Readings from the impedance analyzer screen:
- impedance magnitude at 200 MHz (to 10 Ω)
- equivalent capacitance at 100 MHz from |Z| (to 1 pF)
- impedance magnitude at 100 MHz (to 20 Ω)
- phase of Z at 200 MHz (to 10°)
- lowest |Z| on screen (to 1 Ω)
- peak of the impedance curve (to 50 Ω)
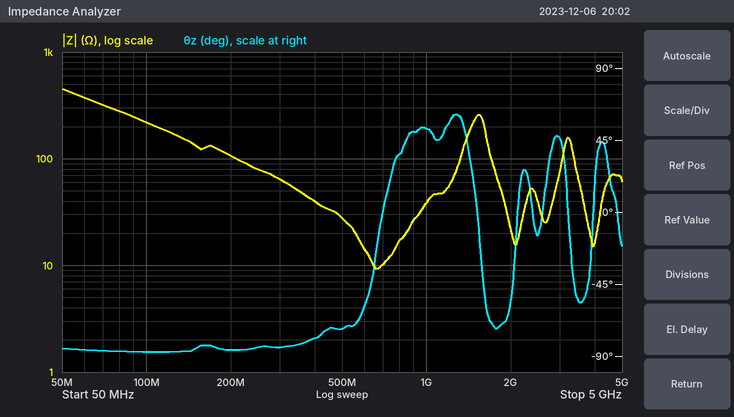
110 Ω
7 pF
220 Ω
-90°
9 Ω
450 Ω
